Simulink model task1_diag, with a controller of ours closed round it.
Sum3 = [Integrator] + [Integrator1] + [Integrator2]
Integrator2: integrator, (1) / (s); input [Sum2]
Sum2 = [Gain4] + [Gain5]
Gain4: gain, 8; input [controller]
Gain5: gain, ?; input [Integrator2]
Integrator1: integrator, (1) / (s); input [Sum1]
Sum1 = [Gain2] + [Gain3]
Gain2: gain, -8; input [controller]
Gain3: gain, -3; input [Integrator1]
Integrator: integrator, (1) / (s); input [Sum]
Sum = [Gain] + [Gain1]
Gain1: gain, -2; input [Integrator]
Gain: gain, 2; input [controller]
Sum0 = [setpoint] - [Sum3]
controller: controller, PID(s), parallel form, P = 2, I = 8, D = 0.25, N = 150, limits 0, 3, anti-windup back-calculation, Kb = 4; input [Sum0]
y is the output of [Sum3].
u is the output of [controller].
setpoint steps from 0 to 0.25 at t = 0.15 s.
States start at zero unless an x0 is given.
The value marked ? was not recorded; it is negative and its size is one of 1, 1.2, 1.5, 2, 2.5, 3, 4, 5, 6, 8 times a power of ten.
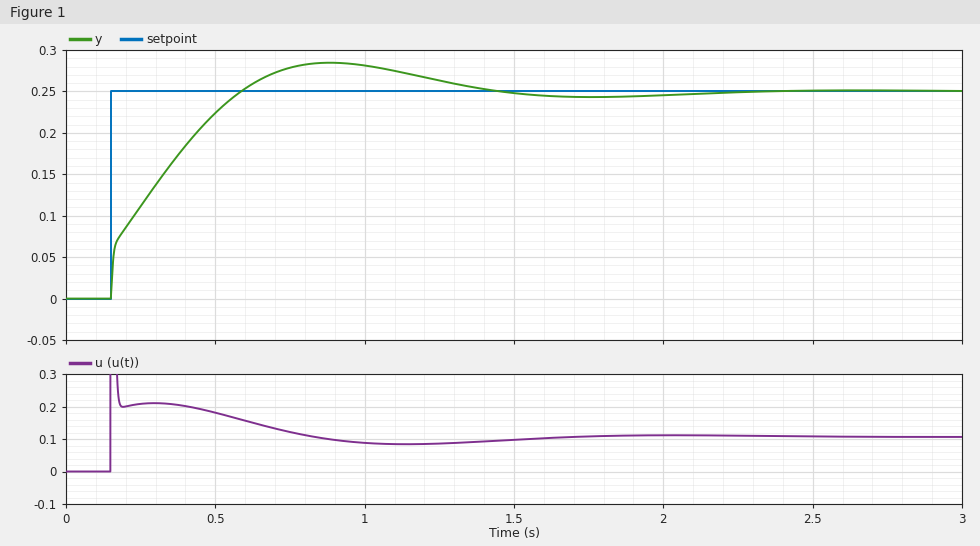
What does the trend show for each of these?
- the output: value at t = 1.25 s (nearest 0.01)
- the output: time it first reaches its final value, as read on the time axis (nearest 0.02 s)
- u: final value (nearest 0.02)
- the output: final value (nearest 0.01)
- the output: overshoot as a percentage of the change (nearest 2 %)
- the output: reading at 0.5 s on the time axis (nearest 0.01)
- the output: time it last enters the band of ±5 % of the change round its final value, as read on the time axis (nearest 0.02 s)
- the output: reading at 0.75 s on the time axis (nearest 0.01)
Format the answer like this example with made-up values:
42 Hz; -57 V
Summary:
0.26; 0.58 s; 0.10; 0.25; 14 %; 0.22; 1.26 s; 0.28
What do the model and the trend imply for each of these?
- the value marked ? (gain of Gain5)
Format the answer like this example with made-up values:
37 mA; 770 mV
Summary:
-2
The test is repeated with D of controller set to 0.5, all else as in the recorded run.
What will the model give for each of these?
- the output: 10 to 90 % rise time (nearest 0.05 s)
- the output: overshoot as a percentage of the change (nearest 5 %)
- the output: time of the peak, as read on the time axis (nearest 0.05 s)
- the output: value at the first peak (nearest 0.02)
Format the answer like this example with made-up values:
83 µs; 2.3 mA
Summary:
0.55 s; 15 %; 1.20 s; 0.28
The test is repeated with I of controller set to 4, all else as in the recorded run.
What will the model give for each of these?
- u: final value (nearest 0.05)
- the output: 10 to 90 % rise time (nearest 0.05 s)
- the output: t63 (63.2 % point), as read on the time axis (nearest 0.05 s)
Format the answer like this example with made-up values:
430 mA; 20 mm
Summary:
0.10; 0.50 s; 0.40 s
